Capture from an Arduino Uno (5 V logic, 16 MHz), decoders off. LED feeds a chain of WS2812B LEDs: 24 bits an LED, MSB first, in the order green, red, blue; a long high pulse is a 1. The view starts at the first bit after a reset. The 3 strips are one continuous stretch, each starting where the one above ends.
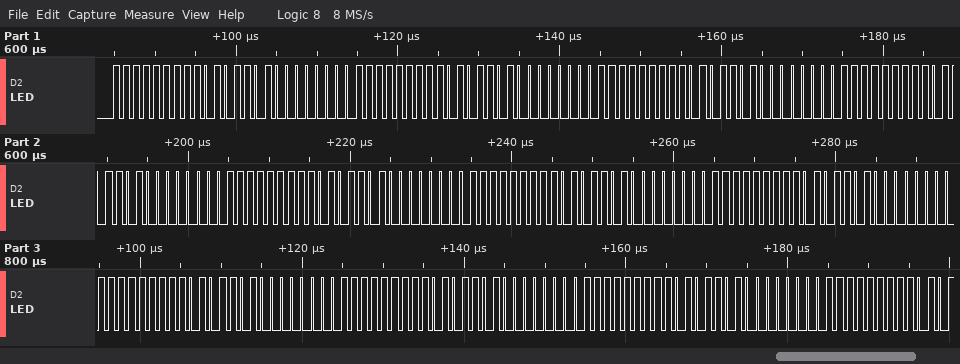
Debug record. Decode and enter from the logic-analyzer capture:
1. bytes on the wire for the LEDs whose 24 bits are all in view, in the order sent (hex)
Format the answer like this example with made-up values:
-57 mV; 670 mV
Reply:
FF AD 00 FF AD 00 FF AD 00 FF AD 00 FF AD 00 FF AD 00 FF AD 00 FF AD 00 FF AD 00 FF AD 00
